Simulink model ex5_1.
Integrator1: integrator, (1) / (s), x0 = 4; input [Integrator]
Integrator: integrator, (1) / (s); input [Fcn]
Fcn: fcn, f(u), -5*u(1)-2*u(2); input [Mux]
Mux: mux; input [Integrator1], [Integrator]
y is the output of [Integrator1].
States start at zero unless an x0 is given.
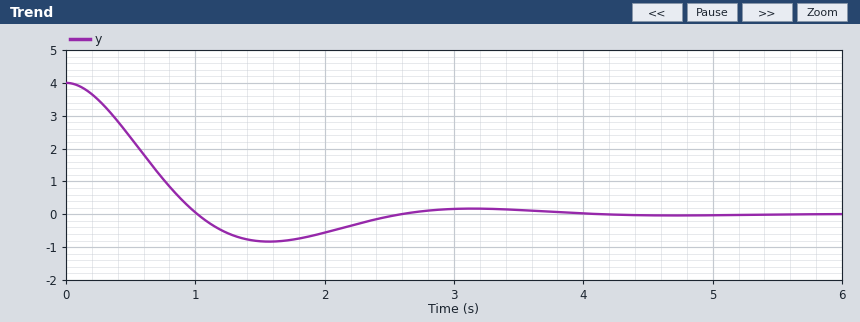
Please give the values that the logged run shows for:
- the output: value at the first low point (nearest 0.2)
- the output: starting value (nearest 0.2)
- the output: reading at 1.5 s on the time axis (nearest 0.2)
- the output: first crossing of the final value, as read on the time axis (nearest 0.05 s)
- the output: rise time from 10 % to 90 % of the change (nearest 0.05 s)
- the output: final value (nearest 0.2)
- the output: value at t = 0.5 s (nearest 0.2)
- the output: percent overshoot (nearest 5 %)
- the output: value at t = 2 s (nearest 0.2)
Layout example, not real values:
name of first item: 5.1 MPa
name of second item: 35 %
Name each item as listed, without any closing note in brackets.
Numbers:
the output: value at the first low point: -0.8
the output: starting value: 4.0
the output: reading at 1.5 s on the time axis: -0.8
the output: first crossing of the final value, as read on the time axis: 1.00 s
the output: rise time from 10 % to 90 % of the change: 0.70 s
the output: final value: 0.0
the output: value at t = 0.5 s: 2.4
the output: percent overshoot: 20 %
the output: value at t = 2 s: -0.6
